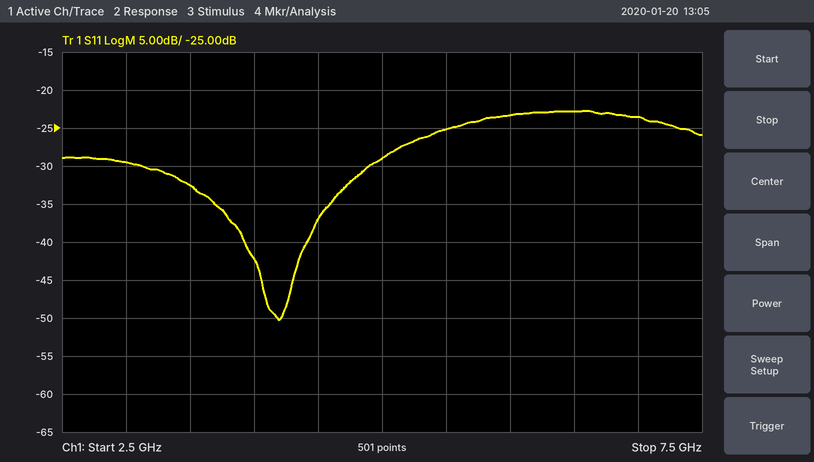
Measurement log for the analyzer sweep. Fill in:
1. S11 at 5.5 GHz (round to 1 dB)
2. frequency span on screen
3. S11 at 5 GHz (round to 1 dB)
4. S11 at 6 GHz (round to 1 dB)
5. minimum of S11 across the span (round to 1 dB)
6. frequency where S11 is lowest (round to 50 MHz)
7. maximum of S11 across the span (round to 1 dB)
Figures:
-25 dB
5 GHz
-29 dB
-23 dB
-50 dB
4.20 GHz
-23 dB
